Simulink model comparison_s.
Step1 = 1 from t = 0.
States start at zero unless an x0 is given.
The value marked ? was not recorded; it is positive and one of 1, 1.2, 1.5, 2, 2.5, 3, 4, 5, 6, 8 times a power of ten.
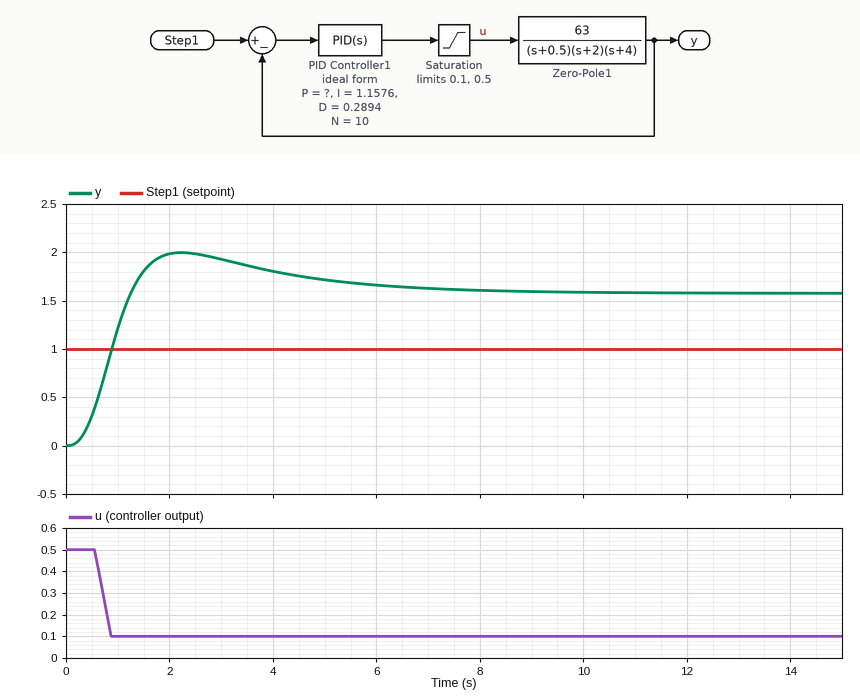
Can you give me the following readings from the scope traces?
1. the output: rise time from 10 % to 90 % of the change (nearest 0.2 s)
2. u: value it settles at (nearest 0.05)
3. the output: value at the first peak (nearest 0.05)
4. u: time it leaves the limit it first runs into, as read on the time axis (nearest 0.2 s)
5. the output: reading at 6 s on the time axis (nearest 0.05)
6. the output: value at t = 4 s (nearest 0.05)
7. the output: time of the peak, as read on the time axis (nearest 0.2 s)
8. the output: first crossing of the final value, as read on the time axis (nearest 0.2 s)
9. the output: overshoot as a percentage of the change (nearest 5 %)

0.8 s
0.10
2.00
0.6 s
1.65
1.80
2.2 s
1.2 s
25 %
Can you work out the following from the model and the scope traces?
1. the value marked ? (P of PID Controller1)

0.6
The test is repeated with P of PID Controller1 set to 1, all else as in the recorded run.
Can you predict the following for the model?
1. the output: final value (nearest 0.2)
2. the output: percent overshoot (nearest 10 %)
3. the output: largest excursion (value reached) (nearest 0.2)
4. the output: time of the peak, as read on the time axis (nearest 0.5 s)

1.6
40 %
2.2
2.0 s
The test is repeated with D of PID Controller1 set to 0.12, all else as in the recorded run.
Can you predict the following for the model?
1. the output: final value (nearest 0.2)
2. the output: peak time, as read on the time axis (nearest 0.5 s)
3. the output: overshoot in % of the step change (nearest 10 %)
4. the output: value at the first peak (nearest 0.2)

1.6
2.0 s
40 %
2.2
